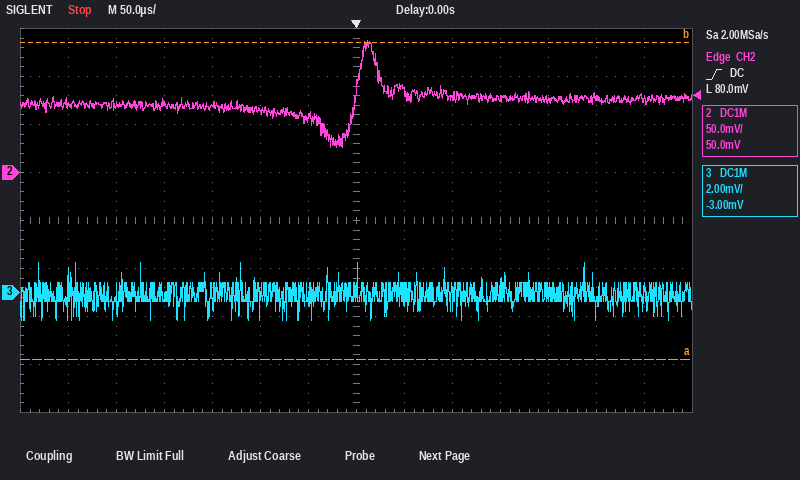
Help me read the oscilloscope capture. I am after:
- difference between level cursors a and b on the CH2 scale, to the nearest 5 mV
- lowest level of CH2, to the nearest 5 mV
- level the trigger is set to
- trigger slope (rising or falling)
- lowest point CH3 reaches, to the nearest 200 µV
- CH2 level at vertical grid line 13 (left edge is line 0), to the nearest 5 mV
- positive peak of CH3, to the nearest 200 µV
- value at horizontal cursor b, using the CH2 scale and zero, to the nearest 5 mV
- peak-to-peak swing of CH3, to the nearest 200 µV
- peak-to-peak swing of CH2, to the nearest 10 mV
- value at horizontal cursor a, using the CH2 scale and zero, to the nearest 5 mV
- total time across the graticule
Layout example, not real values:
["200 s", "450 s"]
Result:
["330 mV", "25 mV", "80.0 mV", "rising", "-1.2 mV", "75 mV", "1.2 mV", "135 mV", "2.4 mV", "110 mV", "-195 mV", "700 µs"]
